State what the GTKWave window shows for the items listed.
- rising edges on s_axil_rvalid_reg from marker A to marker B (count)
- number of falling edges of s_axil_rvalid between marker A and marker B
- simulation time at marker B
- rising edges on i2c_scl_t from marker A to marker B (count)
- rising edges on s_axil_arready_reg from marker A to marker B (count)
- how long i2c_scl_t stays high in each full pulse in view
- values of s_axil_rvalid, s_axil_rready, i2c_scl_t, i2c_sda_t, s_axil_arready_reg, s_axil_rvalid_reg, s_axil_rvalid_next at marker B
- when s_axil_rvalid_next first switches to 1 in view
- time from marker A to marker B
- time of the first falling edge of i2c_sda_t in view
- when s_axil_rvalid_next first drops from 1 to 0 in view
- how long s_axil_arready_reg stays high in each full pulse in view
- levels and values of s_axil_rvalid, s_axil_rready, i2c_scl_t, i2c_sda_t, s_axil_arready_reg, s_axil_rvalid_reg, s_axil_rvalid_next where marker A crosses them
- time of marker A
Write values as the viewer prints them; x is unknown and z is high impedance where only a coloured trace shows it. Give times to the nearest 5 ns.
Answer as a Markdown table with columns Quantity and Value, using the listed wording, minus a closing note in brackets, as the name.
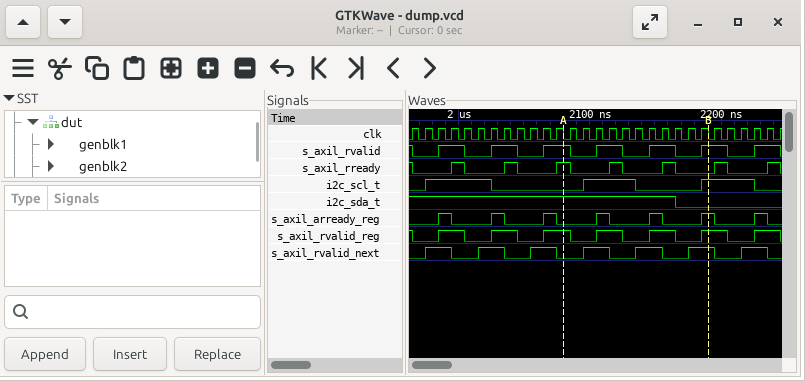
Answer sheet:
| Quantity | Value |
|---|---|
| rising edges on s_axil_rvalid_reg from marker A to marker B | 3 |
| number of falling edges of s_axil_rvalid between marker A and marker B | 3 |
| simulation time at marker B | 2190 ns |
| rising edges on i2c_scl_t from marker A to marker B | 2 |
| rising edges on s_axil_arready_reg from marker A to marker B | 3 |
| how long i2c_scl_t stays high in each full pulse in view | 50 ns, 40 ns, 40 ns |
| values of s_axil_rvalid, s_axil_rready, i2c_scl_t, i2c_sda_t, s_axil_arready_reg, s_axil_rvalid_reg, s_axil_rvalid_next at marker B | s_axil_rvalid=1, s_axil_rready=0, i2c_scl_t=1, i2c_sda_t=0, s_axil_arready_reg=1, s_axil_rvalid_reg=1, s_axil_rvalid_next=1 |
| when s_axil_rvalid_next first switches to 1 in view | 1975 ns |
| time from marker A to marker B | 110 ns |
| time of the first falling edge of i2c_sda_t in view | 2165 ns |
| when s_axil_rvalid_next first drops from 1 to 0 in view | 1995 ns |
| how long s_axil_arready_reg stays high in each full pulse in view | 10 ns, 10 ns, 10 ns, 10 ns, 10 ns, 10 ns, 10 ns |
| levels and values of s_axil_rvalid, s_axil_rready, i2c_scl_t, i2c_sda_t, s_axil_arready_reg, s_axil_rvalid_reg, s_axil_rvalid_next where marker A crosses them | s_axil_rvalid=1, s_axil_rready=1, i2c_scl_t=0, i2c_sda_t=1, s_axil_arready_reg=0, s_axil_rvalid_reg=1, s_axil_rvalid_next=0 |
| time of marker A | 2080 ns |
